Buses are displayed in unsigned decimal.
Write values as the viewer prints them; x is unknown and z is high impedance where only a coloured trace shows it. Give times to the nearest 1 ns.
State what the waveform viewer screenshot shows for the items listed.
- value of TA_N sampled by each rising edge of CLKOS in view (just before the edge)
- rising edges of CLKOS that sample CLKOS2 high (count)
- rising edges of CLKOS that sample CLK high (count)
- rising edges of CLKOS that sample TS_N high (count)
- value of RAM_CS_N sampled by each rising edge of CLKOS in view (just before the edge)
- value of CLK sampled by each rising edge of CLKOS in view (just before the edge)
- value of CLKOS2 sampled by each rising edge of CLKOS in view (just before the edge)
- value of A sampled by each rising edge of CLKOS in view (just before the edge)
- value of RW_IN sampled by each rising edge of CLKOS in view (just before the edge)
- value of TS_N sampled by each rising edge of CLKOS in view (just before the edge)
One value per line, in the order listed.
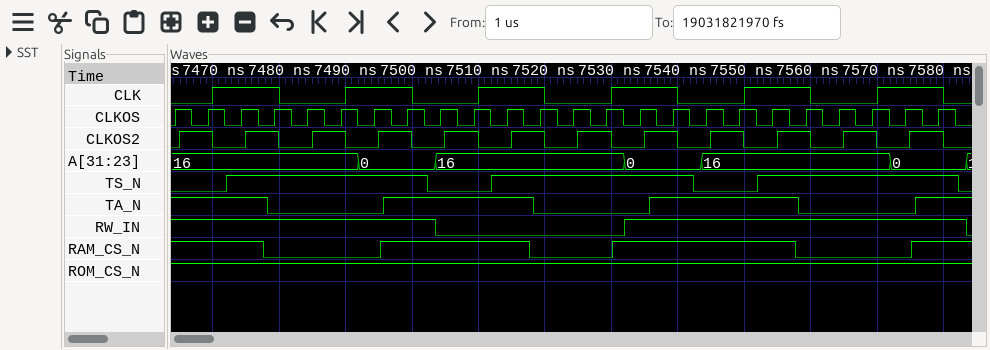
1 1 1 0 0 0 0 1 1 1 1 0 0 0 0 1 1 1 1 0 0 0 0 1
12
12
18
1 1 1 0 0 0 0 1 1 1 1 0 0 0 1 1 1 1 1 0 0 0 0 1
0 0 1 1 0 0 1 1 0 0 1 1 0 0 1 1 0 0 1 1 0 0 1 1
0 1 0 1 0 1 0 1 0 1 0 1 0 1 0 1 0 1 0 1 0 1 0 1
16, 16, 16, 16, 16, 16, 0, 0, 16, 16, 16, 16, 16, 16, 0, 0, 16, 16, 16, 16, 16, 16, 0, 0
1 1 1 1 1 1 1 1 0 0 0 0 0 0 1 1 1 1 1 1 1 1 1 1
0 0 1 1 1 1 1 1 0 0 1 1 1 1 1 1 0 0 1 1 1 1 1 1
